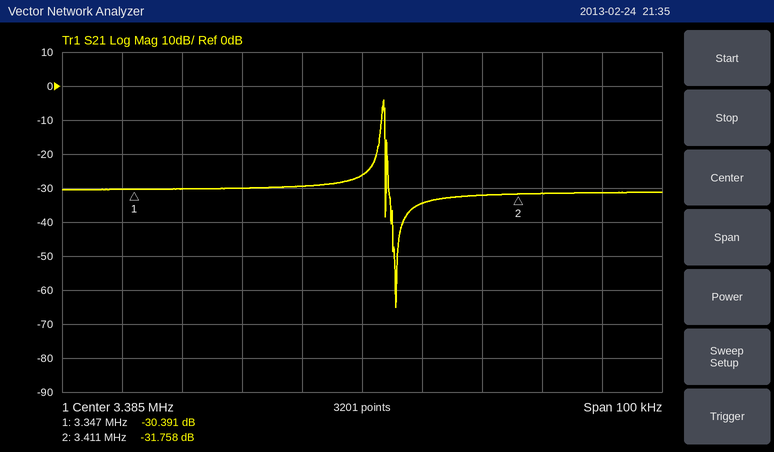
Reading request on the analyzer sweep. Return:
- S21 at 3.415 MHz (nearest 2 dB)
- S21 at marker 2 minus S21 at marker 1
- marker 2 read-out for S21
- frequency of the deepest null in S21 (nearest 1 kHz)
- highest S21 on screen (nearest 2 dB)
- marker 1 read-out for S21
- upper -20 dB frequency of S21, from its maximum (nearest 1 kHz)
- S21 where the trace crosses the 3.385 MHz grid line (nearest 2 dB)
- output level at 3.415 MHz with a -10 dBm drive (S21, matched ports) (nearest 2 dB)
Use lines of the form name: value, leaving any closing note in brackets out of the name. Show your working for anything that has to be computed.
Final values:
S21 at 3.415 MHz: -32 dB
S21 at marker 2 minus S21 at marker 1: -31.758 − (-30.391) = -1.367 dB
marker 2 read-out for S21: -31.758 dB
frequency of the deepest null in S21: 3.391 MHz
highest S21 on screen: -4 dB
marker 1 read-out for S21: -30.391 dB
upper -20 dB frequency of S21, from its maximum: 3.389 MHz
S21 where the trace crosses the 3.385 MHz grid line: -26 dB
output level at 3.415 MHz with a -10 dBm drive (S21, matched ports): -10 dBm + (-32 dB) = -42 dBm
